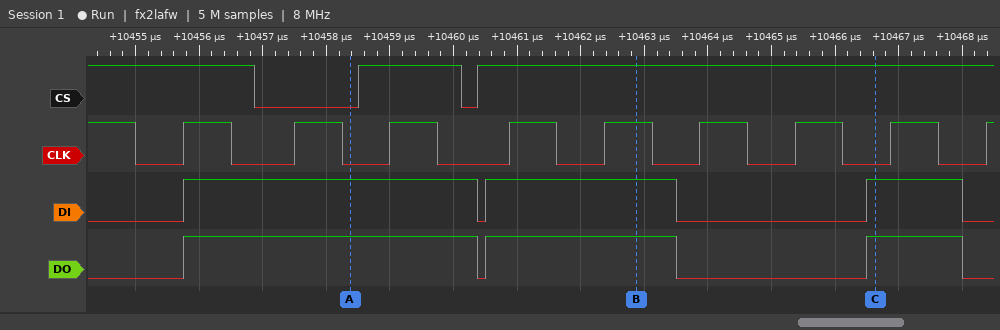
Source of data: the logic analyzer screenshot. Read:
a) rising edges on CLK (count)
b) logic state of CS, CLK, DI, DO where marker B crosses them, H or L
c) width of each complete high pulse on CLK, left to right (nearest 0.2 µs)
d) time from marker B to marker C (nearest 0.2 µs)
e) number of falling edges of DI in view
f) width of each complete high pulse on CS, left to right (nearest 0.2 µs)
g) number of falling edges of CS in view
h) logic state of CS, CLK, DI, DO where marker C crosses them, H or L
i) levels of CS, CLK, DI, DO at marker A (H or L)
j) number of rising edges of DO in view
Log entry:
9
CS=H, CLK=H, DI=H, DO=H
0.8 µs, 0.8 µs, 0.8 µs, 0.8 µs, 0.8 µs, 0.8 µs, 0.8 µs, 0.8 µs
3.8 µs
3
1.6 µs
2
CS=H, CLK=L, DI=H, DO=H
CS=L, CLK=L, DI=H, DO=H
3
